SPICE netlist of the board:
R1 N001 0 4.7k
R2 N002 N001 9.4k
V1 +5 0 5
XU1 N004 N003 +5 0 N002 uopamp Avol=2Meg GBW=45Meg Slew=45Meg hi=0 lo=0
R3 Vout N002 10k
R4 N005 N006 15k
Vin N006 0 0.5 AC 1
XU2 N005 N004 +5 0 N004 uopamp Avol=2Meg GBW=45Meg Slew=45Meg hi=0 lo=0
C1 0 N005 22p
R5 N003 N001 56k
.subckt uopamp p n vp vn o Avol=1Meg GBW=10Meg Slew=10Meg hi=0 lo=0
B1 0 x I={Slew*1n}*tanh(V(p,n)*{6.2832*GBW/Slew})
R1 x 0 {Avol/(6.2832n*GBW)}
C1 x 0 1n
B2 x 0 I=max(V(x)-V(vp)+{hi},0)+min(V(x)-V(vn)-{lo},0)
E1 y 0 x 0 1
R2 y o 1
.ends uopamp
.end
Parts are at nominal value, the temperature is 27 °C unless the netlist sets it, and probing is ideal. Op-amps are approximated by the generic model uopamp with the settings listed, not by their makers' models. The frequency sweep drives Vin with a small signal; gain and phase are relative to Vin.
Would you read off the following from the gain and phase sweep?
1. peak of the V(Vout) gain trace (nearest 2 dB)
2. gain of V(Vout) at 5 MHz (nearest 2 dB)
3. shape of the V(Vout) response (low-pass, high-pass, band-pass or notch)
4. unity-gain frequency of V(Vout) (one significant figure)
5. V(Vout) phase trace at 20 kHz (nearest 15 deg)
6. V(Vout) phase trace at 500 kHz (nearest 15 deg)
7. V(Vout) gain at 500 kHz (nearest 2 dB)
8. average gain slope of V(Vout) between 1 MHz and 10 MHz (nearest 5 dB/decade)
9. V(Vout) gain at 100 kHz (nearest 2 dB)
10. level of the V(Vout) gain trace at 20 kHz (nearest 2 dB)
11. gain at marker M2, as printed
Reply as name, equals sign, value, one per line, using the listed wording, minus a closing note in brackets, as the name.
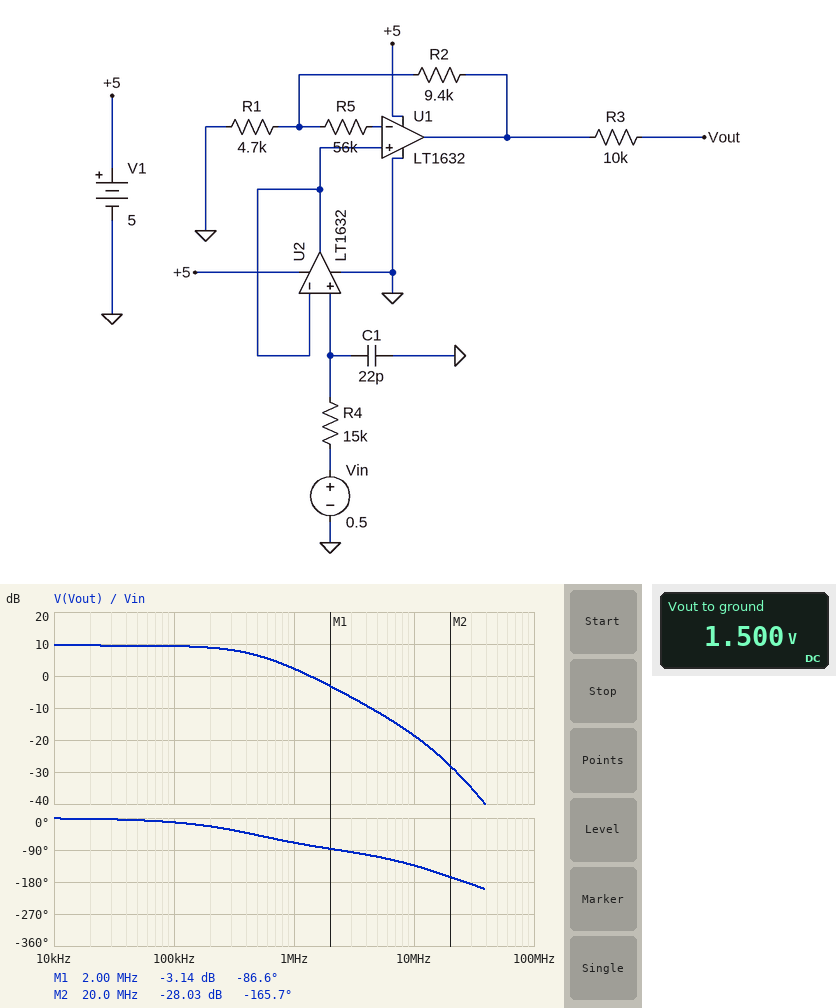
peak of the V(Vout) gain trace = 10 dB
gain of V(Vout) at 5 MHz = -12 dB
shape of the V(Vout) response = low-pass
unity-gain frequency of V(Vout) = 1 MHz
V(Vout) phase trace at 20 kHz = 0 deg
V(Vout) phase trace at 500 kHz = -45 deg
V(Vout) gain at 500 kHz = 6 dB
average gain slope of V(Vout) between 1 MHz and 10 MHz = -20 dB/decade
V(Vout) gain at 100 kHz = 10 dB
level of the V(Vout) gain trace at 20 kHz = 10 dB
gain at marker M2, as printed = -28.03 dB
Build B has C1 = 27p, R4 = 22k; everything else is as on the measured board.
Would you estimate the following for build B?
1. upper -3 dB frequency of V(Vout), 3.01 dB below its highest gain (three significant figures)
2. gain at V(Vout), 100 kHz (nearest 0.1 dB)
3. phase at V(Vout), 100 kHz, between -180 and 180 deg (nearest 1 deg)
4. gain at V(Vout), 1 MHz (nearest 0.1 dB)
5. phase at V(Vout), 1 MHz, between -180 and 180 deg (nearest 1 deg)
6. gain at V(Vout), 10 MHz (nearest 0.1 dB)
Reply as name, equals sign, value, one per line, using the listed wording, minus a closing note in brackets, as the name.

upper -3 dB frequency of V(Vout), 3.01 dB below its highest gain = 268 kHz
gain at V(Vout), 100 kHz = 9.0 dB
phase at V(Vout), 100 kHz, between -180 and 180 deg = -21 deg
gain at V(Vout), 1 MHz = -2.2 dB
phase at V(Vout), 1 MHz, between -180 and 180 deg = -80 deg
gain at V(Vout), 10 MHz = -23.7 dB
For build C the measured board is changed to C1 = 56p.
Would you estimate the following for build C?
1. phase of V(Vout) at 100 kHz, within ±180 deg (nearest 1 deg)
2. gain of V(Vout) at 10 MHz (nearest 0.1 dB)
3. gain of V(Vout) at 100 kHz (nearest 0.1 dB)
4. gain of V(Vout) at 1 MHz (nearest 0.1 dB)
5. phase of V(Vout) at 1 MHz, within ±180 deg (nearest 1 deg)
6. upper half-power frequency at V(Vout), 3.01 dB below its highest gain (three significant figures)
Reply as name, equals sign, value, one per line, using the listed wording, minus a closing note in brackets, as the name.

phase of V(Vout) at 100 kHz, within ±180 deg = -28 deg
gain of V(Vout) at 10 MHz = -26.7 dB
gain of V(Vout) at 100 kHz = 8.5 dB
gain of V(Vout) at 1 MHz = -5.1 dB
phase of V(Vout) at 1 MHz, within ±180 deg = -84 deg
upper half-power frequency at V(Vout), 3.01 dB below its highest gain = 189 kHz
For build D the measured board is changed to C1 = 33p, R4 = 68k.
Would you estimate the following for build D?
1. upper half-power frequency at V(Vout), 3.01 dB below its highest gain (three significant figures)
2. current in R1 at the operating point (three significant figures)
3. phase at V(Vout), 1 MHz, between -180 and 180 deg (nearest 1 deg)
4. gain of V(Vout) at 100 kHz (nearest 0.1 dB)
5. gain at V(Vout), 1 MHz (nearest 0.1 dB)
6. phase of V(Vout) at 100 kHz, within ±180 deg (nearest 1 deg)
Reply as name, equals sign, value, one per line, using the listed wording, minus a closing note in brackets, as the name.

upper half-power frequency at V(Vout), 3.01 dB below its highest gain = 70.9 kHz
current in R1 at the operating point = 106 µA
phase at V(Vout), 1 MHz, between -180 and 180 deg = -91 deg
gain of V(Vout) at 100 kHz = 4.8 dB
gain at V(Vout), 1 MHz = -13.5 dB
phase of V(Vout) at 100 kHz, within ±180 deg = -55 deg
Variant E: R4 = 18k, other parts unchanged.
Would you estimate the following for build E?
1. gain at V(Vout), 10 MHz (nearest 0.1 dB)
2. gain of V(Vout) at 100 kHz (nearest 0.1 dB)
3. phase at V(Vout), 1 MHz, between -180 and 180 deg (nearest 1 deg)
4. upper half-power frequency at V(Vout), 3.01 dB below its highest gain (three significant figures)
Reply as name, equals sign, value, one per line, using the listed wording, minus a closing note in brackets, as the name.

gain at V(Vout), 10 MHz = -20.2 dB
gain of V(Vout) at 100 kHz = 9.3 dB
phase at V(Vout), 1 MHz, between -180 and 180 deg = -73 deg
upper half-power frequency at V(Vout), 3.01 dB below its highest gain = 402 kHz
